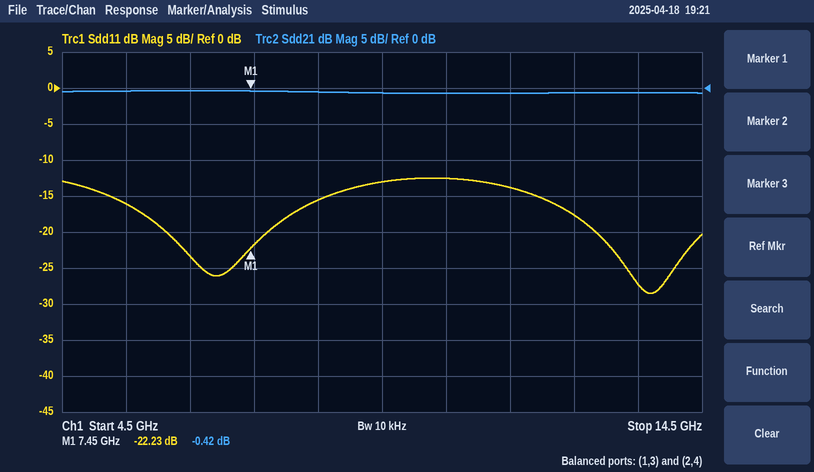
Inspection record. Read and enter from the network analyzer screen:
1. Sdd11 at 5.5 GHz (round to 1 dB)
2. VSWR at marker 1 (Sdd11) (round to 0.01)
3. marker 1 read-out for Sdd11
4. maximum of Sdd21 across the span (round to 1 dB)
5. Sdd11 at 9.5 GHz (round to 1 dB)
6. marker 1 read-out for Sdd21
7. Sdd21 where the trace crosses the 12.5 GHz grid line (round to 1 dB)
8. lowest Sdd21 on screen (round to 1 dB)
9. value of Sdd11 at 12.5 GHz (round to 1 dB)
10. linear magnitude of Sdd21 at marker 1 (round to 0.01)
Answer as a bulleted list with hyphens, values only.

- -16 dB
- 1.17
- -22.23 dB
- 0 dB
- -13 dB
- -0.42 dB
- -1 dB
- -1 dB
- -18 dB
- 0.95
